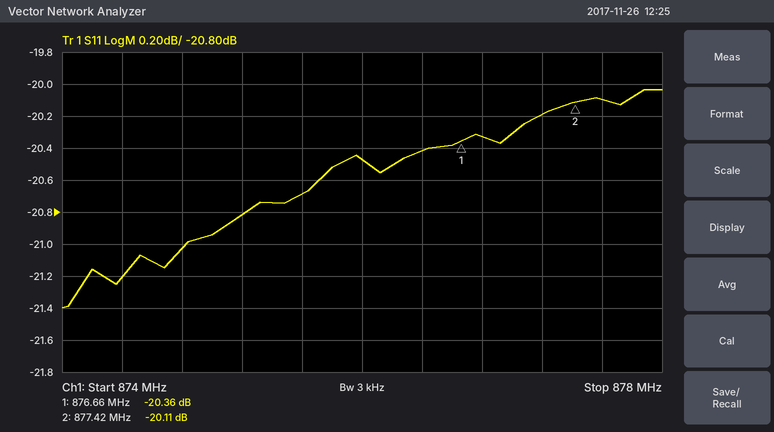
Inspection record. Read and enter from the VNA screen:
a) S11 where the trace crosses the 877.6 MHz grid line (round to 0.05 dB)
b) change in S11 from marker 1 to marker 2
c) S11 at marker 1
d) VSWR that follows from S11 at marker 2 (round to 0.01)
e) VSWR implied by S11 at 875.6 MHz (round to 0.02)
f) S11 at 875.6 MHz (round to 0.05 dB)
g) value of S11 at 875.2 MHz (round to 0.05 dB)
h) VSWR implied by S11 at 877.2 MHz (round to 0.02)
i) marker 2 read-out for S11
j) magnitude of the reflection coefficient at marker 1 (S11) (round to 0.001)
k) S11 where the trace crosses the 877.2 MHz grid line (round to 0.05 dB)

-20.10 dB
0.25 dB
-20.36 dB
1.22
1.20
-20.70 dB
-20.80 dB
1.22
-20.11 dB
0.096
-20.20 dB
